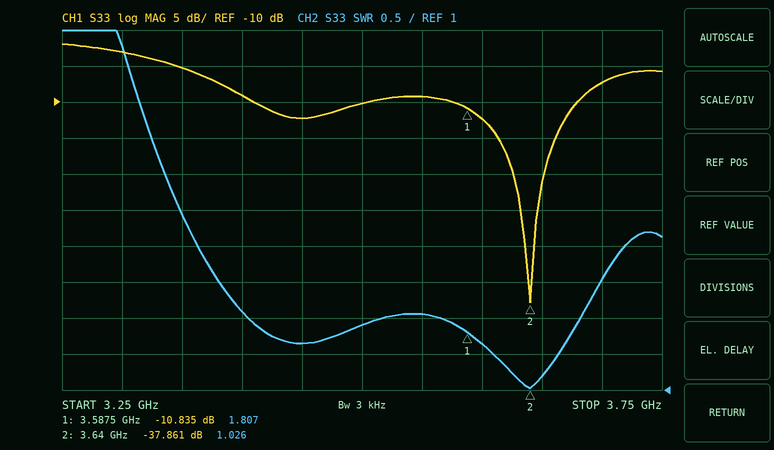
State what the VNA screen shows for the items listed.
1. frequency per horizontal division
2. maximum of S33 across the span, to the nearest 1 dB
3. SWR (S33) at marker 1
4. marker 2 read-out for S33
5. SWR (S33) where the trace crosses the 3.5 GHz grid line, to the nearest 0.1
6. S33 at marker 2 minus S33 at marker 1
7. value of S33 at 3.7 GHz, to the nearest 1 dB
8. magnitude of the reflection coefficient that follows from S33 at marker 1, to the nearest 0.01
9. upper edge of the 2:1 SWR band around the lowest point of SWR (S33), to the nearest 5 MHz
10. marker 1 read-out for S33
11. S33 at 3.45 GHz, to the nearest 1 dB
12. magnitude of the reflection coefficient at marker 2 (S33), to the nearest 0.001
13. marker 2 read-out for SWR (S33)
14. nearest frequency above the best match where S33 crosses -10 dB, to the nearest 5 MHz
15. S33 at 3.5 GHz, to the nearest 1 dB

50 MHz
-2 dB
1.807
-37.861 dB
1.9
-27.026 dB
-7 dB
0.29
3.680 GHz
-10.835 dB
-12 dB
0.013
1.026
3.680 GHz
-10 dB
